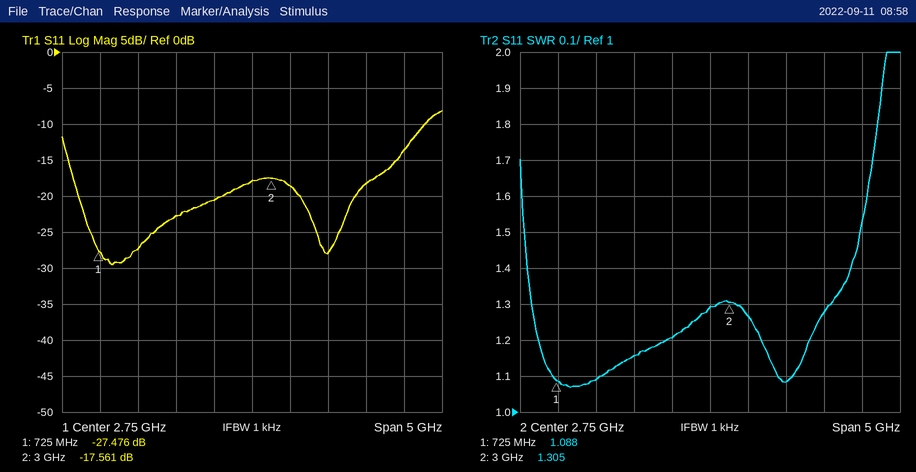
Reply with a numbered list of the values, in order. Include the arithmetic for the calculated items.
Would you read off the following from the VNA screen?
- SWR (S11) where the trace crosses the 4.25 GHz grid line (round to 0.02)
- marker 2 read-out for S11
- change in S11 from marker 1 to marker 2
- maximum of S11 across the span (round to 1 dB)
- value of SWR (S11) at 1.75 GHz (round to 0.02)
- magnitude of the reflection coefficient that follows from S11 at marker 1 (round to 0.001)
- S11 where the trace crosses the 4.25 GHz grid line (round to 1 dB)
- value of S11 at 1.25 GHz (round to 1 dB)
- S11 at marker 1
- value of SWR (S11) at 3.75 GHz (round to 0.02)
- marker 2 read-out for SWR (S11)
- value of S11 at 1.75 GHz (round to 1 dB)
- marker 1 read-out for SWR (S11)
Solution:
1. 1.28
2. -17.561 dB
3. -17.561 − (-27.476) = 9.915 dB
4. -8 dB
5. 1.16
6. 10^(-27.476/20) ≈ 0.042
7. -18 dB
8. -27 dB
9. -27.476 dB
10. 1.08
11. 1.305
12. -23 dB
13. 1.088
